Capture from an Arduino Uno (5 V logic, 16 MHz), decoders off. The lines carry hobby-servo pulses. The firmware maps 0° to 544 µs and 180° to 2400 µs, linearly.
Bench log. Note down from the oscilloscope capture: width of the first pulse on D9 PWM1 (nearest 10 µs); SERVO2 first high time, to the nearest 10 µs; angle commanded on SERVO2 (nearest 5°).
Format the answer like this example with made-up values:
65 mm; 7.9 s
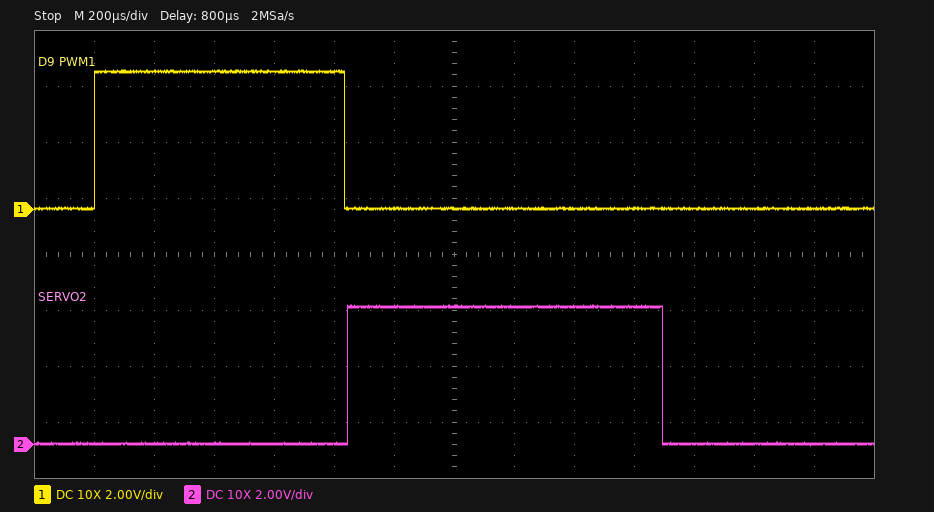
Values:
830 µs; 1050 µs; 50°
